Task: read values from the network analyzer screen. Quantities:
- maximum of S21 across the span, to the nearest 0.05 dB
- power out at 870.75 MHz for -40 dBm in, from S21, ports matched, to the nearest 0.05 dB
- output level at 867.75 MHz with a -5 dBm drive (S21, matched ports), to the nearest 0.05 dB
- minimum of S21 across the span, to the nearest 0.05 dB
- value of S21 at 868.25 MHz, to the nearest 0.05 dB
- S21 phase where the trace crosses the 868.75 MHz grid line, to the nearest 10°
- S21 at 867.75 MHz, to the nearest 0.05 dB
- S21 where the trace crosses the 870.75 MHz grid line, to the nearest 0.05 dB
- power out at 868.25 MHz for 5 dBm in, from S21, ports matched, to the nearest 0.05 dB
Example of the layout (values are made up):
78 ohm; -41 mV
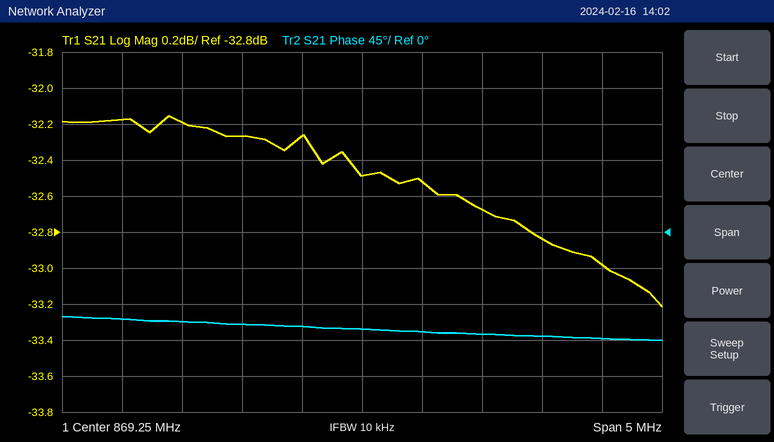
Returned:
-32.15 dB; -72.85 dBm; -37.20 dBm; -33.20 dB; -32.25 dB; -120°; -32.20 dB; -32.85 dB; -27.25 dBm
